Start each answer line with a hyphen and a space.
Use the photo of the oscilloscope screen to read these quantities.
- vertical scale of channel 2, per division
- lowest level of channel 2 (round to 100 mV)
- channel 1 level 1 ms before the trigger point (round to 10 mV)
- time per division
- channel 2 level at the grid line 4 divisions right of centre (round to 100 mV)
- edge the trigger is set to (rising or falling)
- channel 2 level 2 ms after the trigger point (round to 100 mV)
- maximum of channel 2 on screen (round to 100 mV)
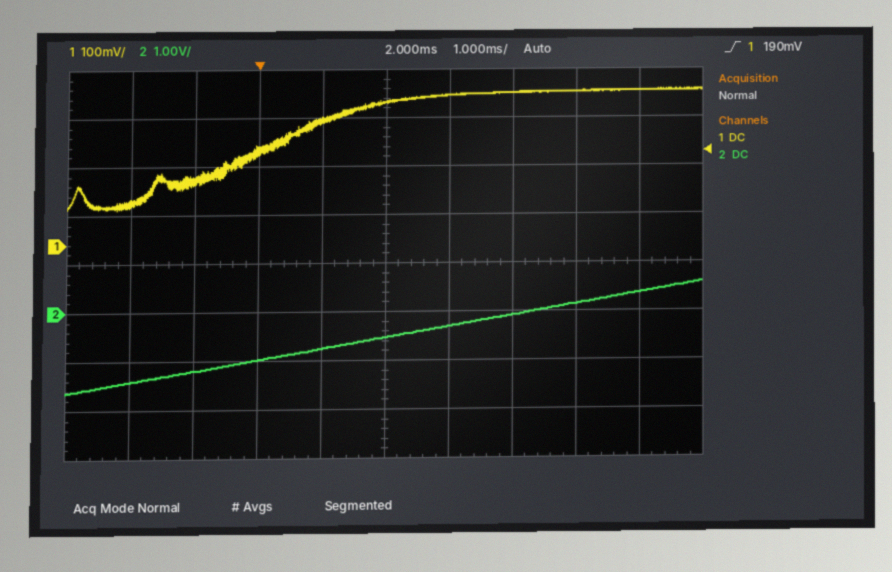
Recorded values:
- 1 V
- -1.6 V
- 130 mV
- 1 ms
- 400 mV
- rising
- -500 mV
- 600 mV
